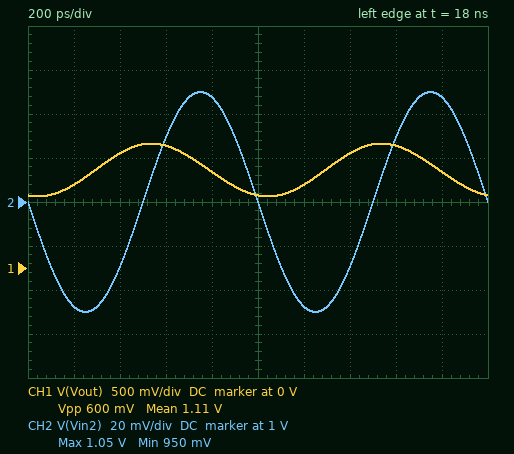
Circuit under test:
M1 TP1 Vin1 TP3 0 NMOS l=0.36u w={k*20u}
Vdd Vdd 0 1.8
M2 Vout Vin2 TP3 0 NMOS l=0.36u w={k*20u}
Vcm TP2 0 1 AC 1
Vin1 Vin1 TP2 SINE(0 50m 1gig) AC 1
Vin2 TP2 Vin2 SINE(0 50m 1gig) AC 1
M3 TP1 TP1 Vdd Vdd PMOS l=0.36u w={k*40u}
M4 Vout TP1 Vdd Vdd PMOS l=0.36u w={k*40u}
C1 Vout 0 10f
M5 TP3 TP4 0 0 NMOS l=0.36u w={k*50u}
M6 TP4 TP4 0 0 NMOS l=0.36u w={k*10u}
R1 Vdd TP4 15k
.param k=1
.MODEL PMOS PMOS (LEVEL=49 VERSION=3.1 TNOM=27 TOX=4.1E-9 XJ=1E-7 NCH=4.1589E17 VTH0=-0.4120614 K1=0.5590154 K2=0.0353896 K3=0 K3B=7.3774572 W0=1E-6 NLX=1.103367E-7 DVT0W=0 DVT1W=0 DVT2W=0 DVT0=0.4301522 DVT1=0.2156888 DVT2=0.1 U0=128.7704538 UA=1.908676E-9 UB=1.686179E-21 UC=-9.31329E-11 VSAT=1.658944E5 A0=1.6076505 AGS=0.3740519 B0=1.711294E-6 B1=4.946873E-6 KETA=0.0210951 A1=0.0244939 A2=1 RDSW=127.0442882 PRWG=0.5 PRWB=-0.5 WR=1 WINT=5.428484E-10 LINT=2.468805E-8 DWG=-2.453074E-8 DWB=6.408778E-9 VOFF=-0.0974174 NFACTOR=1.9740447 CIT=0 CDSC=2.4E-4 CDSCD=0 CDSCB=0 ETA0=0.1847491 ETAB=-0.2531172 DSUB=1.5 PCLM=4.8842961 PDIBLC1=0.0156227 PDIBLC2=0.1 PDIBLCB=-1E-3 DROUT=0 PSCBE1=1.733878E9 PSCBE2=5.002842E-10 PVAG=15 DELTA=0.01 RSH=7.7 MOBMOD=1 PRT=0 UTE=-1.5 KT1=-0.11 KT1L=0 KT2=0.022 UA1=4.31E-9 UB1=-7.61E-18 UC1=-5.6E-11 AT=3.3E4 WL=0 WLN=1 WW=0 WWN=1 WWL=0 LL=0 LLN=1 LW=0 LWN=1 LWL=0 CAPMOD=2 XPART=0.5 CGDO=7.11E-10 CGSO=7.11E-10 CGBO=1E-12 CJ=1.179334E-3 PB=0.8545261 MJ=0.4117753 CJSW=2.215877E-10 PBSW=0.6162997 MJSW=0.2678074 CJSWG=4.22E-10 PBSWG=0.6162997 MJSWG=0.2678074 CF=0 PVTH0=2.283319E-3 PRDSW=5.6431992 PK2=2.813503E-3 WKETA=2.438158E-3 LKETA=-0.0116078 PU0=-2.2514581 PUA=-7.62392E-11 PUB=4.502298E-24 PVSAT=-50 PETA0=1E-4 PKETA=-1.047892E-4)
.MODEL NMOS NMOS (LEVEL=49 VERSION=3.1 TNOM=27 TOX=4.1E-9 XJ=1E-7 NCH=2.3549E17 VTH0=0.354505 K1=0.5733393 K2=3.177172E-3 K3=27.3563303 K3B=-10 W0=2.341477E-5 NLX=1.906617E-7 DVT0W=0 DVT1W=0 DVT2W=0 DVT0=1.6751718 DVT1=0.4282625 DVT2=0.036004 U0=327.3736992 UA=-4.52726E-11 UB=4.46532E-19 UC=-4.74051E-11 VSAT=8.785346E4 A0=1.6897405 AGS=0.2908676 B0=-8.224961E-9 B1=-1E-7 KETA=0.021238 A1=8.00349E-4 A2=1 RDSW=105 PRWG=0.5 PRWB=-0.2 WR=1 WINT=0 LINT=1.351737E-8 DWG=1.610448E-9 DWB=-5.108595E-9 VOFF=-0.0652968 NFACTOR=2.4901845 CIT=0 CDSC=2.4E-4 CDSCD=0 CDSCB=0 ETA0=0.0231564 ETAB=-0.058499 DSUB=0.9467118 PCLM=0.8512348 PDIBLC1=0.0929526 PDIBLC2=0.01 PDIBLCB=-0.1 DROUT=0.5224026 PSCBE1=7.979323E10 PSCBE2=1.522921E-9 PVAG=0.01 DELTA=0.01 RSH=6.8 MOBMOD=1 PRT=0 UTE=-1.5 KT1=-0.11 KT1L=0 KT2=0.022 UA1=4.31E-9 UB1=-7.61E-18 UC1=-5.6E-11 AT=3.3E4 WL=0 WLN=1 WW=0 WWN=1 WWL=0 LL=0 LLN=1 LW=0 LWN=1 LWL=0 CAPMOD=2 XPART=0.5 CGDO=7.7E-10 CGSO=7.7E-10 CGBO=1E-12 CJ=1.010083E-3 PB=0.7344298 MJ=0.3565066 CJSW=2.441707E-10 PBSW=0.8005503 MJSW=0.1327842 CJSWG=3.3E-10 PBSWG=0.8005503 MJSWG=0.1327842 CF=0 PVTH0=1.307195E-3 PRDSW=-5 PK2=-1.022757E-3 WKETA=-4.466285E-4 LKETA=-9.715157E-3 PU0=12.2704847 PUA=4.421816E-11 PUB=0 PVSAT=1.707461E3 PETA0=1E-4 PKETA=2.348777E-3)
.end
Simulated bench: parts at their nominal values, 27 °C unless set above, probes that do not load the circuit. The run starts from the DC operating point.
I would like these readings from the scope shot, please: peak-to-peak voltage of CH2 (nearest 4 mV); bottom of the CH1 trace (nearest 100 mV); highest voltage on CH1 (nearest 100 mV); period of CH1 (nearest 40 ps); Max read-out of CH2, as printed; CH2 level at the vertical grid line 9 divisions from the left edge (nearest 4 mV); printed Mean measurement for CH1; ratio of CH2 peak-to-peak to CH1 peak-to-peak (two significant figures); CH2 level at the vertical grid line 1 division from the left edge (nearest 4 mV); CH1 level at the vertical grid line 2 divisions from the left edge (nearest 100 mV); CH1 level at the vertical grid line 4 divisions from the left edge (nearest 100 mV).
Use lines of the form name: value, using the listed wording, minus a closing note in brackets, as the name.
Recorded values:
peak-to-peak voltage of CH2: 100 mV
bottom of the CH1 trace: 800 mV
highest voltage on CH1: 1.4 V
period of CH1: 1.00 ns
Max read-out of CH2, as printed: 1.05 V
CH2 level at the vertical grid line 9 divisions from the left edge: 1.048 V
printed Mean measurement for CH1: 1.11 V
ratio of CH2 peak-to-peak to CH1 peak-to-peak: 0.17
CH2 level at the vertical grid line 1 division from the left edge: 952 mV
CH1 level at the vertical grid line 2 divisions from the left edge: 1.3 V
CH1 level at the vertical grid line 4 divisions from the left edge: 1.1 V
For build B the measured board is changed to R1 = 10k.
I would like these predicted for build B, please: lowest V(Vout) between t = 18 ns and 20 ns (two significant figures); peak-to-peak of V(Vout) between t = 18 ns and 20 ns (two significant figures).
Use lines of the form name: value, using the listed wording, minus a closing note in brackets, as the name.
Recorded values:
lowest V(Vout) between t = 18 ns and 20 ns: 700 mV
peak-to-peak of V(Vout) between t = 18 ns and 20 ns: 740 mV
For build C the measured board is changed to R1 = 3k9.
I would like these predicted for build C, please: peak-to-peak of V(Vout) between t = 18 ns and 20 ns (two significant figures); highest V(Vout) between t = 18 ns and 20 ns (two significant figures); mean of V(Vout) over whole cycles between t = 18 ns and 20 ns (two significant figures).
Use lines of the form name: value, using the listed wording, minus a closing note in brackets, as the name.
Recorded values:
peak-to-peak of V(Vout) between t = 18 ns and 20 ns: 990 mV
highest V(Vout) between t = 18 ns and 20 ns: 1.5 V
mean of V(Vout) over whole cycles between t = 18 ns and 20 ns: 960 mV
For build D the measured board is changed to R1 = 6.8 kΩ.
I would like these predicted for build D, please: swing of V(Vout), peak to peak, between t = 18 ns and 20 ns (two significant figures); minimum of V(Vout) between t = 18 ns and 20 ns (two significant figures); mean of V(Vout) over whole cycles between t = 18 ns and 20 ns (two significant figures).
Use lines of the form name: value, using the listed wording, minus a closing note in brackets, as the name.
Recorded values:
swing of V(Vout), peak to peak, between t = 18 ns and 20 ns: 870 mV
minimum of V(Vout) between t = 18 ns and 20 ns: 590 mV
mean of V(Vout) over whole cycles between t = 18 ns and 20 ns: 1.0 V
